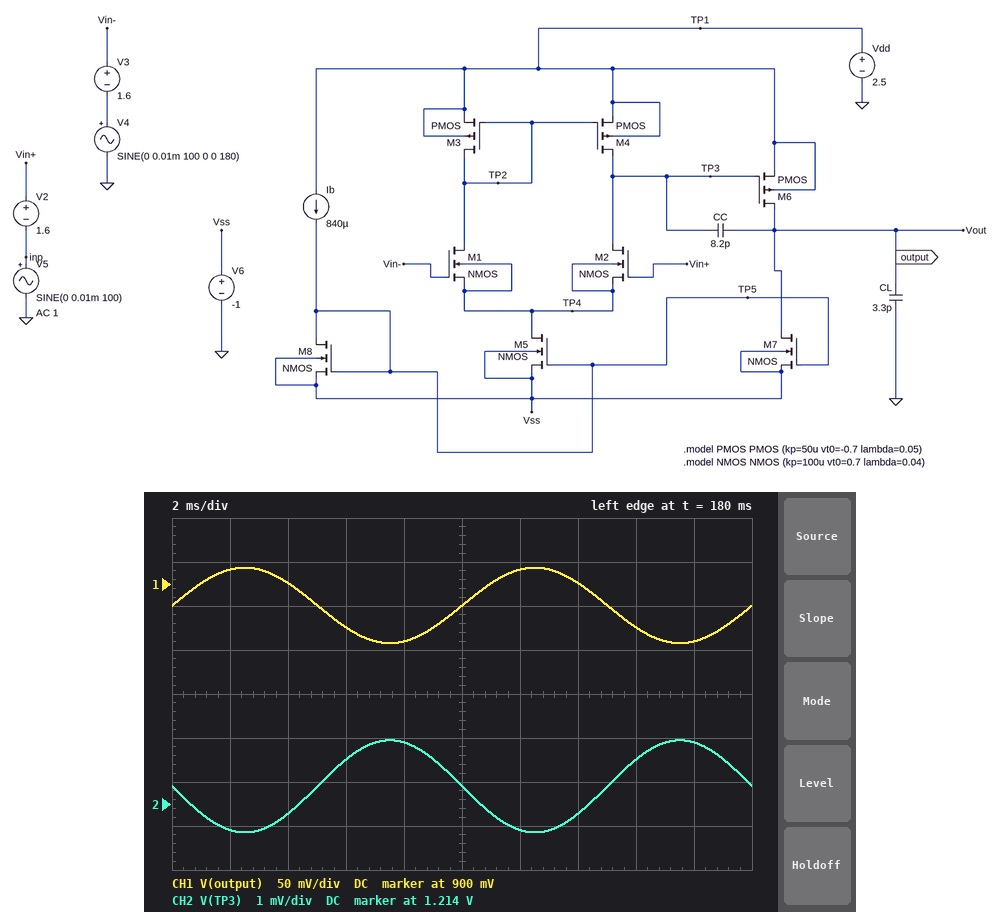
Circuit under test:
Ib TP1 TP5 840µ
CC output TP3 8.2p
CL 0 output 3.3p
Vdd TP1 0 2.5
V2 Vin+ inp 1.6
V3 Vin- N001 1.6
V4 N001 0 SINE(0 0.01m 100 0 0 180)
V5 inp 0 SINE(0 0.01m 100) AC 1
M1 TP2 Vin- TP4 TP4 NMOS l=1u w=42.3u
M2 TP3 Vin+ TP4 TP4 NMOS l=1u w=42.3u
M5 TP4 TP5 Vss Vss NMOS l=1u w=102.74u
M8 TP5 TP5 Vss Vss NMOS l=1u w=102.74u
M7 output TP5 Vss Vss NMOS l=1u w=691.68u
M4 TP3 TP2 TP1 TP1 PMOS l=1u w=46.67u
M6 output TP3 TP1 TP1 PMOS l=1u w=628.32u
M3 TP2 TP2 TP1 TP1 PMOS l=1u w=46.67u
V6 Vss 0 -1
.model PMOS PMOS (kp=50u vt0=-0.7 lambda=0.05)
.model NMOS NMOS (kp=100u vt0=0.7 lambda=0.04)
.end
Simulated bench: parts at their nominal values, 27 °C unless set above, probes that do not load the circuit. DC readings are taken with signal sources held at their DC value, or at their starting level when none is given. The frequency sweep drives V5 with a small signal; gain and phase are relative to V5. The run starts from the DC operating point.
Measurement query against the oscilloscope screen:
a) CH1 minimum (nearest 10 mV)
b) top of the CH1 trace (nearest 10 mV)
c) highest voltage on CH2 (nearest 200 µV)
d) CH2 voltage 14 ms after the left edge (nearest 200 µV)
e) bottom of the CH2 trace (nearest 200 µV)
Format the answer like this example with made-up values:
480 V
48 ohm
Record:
830 mV
920 mV
1.2154 V
1.2138 V
1.2134 V
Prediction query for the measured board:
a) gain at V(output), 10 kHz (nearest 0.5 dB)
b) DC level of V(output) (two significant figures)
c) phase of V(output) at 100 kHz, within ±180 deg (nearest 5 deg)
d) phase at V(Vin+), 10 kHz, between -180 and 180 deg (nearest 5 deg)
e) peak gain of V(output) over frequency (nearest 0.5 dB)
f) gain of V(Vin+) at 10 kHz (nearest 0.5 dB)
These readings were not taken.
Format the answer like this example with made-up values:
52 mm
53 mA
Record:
65.5 dB
880 mV
-80 deg
0 deg
66.5 dB
0 dB
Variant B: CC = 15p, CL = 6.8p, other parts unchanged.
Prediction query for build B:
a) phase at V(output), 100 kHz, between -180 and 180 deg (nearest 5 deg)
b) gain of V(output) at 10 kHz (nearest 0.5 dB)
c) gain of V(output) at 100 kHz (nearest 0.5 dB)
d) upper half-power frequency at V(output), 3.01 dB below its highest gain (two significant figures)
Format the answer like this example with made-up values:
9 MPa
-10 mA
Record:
-85 deg
63.0 dB
46.0 dB
9.2 kHz
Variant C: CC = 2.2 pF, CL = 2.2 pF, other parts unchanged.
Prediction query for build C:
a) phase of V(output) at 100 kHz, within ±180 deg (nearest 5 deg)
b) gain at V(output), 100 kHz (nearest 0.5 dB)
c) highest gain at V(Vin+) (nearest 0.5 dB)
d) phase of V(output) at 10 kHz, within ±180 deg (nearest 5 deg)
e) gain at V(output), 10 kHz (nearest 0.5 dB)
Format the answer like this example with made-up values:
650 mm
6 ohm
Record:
-60 deg
61.0 dB
0 dB
-10 deg
66.5 dB
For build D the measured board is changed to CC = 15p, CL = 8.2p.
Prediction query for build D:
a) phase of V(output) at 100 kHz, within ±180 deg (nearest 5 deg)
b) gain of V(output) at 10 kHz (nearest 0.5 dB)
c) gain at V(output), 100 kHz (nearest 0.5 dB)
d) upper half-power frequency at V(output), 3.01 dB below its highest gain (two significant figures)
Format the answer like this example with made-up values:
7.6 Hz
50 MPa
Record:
-85 deg
63.0 dB
46.0 dB
9.2 kHz
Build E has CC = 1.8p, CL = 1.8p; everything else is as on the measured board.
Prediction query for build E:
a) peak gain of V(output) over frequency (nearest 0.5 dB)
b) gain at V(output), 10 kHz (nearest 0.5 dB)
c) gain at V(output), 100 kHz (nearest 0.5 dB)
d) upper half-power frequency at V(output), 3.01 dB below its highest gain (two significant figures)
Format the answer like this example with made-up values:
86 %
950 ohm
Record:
66.5 dB
66.5 dB
62.5 dB
76 kHz
